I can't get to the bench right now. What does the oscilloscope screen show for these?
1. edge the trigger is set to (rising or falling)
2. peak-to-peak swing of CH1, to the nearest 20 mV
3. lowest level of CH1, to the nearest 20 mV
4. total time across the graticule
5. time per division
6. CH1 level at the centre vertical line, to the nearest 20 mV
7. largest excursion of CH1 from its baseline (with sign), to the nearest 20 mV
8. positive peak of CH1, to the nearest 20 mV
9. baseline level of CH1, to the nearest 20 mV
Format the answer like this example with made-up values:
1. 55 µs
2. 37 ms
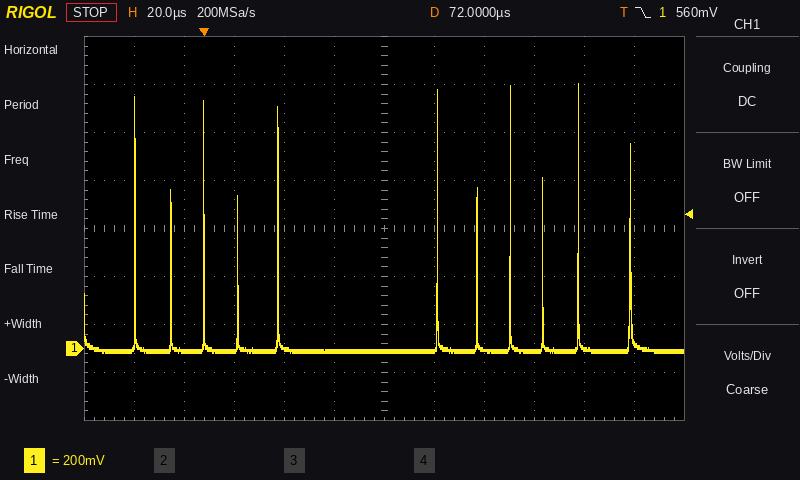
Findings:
1. falling
2. 1.12 V
3. -20 mV
4. 240 µs
5. 20 µs
6. -20 mV
7. +1.12 V
8. 1.10 V
9. -20 mV
